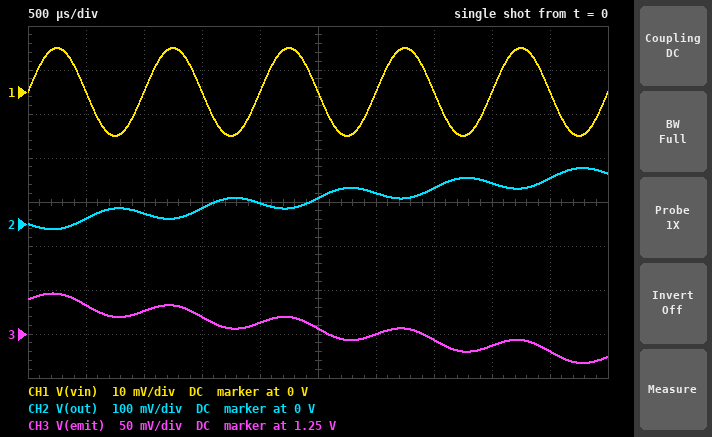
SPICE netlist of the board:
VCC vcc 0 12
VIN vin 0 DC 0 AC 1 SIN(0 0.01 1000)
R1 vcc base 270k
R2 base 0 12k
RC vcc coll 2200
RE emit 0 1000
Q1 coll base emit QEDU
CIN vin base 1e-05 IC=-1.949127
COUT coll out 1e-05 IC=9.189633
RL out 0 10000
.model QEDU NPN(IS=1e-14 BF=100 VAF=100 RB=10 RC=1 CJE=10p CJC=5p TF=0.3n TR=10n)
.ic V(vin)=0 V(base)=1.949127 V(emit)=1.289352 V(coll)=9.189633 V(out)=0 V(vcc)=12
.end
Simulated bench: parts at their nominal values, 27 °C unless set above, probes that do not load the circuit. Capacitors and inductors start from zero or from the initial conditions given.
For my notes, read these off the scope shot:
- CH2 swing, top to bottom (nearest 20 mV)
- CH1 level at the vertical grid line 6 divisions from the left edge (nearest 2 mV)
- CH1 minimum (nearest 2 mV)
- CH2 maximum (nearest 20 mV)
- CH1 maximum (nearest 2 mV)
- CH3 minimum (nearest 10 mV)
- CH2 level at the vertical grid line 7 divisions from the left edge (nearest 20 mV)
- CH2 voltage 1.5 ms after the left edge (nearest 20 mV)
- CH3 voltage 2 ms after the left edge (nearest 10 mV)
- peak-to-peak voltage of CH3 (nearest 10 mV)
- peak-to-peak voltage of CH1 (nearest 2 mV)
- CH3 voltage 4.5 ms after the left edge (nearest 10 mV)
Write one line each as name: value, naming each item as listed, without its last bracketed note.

CH2 swing, top to bottom: 140 mV
CH1 level at the vertical grid line 6 divisions from the left edge: 0 V
CH1 minimum: -10 mV
CH2 maximum: 120 mV
CH1 maximum: 10 mV
CH3 minimum: 1.22 V
CH2 level at the vertical grid line 7 divisions from the left edge: 80 mV
CH2 voltage 1.5 ms after the left edge: 40 mV
CH3 voltage 2 ms after the left edge: 1.26 V
peak-to-peak voltage of CH3: 80 mV
peak-to-peak voltage of CH1: 20 mV
CH3 voltage 4.5 ms after the left edge: 1.23 V
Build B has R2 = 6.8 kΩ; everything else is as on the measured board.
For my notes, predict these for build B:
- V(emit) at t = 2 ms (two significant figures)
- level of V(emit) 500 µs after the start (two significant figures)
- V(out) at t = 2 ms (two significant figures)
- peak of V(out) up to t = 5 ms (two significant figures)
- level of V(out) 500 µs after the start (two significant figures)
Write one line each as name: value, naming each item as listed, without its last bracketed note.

V(emit) at t = 2 ms: 1.2 V
level of V(emit) 500 µs after the start: 1.3 V
V(out) at t = 2 ms: 89 mV
peak of V(out) up to t = 5 ms: 220 mV
level of V(out) 500 µs after the start: 23 mV
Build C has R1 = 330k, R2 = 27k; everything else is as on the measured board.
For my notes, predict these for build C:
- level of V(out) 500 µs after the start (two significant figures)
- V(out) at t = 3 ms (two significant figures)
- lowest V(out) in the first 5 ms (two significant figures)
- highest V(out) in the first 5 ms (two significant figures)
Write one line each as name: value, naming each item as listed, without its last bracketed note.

level of V(out) 500 µs after the start: 4.7 mV
V(out) at t = 3 ms: 28 mV
lowest V(out) in the first 5 ms: -15 mV
highest V(out) in the first 5 ms: 61 mV
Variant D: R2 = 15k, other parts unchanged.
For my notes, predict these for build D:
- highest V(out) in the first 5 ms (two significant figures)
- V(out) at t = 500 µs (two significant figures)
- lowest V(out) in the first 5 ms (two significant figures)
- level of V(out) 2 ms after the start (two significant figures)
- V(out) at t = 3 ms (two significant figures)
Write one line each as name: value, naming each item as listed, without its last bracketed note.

highest V(out) in the first 5 ms: 100 mV
V(out) at t = 500 µs: 9.2 mV
lowest V(out) in the first 5 ms: -13 mV
level of V(out) 2 ms after the start: 36 mV
V(out) at t = 3 ms: 54 mV
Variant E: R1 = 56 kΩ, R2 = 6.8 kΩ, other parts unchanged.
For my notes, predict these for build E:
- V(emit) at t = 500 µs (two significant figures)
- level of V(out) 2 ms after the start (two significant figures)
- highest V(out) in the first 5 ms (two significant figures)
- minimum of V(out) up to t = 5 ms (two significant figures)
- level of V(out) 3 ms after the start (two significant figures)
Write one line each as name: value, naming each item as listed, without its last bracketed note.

V(emit) at t = 500 µs: 1.3 V
level of V(out) 2 ms after the start: 41 mV
highest V(out) in the first 5 ms: 110 mV
minimum of V(out) up to t = 5 ms: -13 mV
level of V(out) 3 ms after the start: 60 mV
